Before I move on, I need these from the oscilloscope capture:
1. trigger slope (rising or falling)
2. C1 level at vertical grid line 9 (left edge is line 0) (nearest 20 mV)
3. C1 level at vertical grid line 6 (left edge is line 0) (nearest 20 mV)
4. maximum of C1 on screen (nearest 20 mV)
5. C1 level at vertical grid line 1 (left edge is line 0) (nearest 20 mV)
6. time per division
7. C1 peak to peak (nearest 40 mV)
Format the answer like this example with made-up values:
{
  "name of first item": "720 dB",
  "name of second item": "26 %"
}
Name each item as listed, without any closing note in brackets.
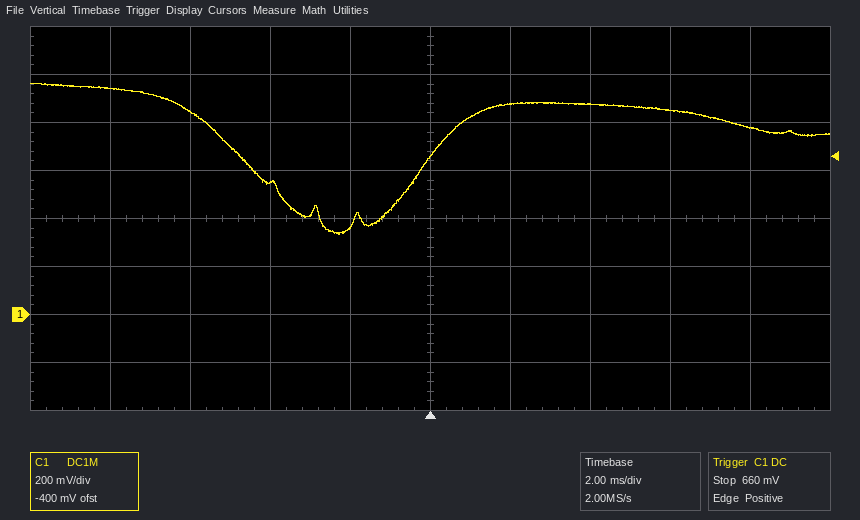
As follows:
{
  "trigger slope": "rising",
  "C1 level at vertical grid line 9 (left edge is line 0)": "780 mV",
  "C1 level at vertical grid line 6 (left edge is line 0)": "880 mV",
  "maximum of C1 on screen": "960 mV",
  "C1 level at vertical grid line 1 (left edge is line 0)": "940 mV",
  "time per division": "2 ms",
  "C1 peak to peak": "640 mV"
}
